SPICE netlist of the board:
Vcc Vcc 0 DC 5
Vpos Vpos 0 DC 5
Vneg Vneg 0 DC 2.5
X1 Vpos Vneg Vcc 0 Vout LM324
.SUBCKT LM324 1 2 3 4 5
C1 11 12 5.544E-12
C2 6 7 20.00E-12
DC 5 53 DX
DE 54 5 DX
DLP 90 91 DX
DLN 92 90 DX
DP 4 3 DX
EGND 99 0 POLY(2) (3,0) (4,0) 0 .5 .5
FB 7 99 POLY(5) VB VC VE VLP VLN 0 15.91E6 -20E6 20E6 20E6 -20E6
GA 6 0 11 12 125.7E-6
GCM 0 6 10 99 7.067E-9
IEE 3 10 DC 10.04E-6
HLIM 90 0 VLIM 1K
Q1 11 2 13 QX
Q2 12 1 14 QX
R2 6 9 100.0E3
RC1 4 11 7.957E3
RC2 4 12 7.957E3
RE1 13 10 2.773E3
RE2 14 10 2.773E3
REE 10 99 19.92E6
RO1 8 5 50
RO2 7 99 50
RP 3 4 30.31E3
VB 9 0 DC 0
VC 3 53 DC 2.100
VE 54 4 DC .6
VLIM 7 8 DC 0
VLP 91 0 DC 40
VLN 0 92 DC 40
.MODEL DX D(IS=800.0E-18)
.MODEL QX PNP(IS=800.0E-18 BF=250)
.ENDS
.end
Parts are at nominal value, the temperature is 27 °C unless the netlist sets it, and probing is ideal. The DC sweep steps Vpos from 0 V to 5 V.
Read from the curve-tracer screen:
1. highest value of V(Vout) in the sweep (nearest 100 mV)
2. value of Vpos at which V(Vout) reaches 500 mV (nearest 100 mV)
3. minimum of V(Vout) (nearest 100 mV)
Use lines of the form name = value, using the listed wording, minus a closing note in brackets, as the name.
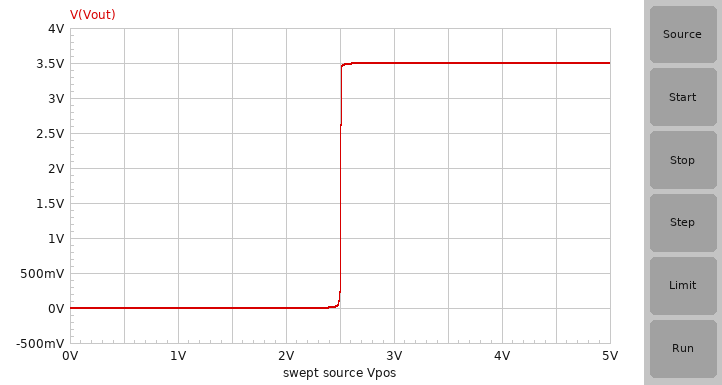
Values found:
highest value of V(Vout) in the sweep = 3.5 V
value of Vpos at which V(Vout) reaches 500 mV = 2.5 V
minimum of V(Vout) = 0 V
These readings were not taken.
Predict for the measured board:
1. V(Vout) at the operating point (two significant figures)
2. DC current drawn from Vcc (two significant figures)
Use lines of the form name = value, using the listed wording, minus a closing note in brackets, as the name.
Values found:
V(Vout) at the operating point = 3.5 V
DC current drawn from Vcc = 170 µA
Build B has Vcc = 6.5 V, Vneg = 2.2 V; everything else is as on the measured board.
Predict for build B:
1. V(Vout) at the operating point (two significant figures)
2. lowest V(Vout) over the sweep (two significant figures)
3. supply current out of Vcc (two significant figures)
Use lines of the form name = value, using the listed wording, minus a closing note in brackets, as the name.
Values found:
V(Vout) at the operating point = 5.0 V
lowest V(Vout) over the sweep = 4.3 mV
supply current out of Vcc = 220 µA
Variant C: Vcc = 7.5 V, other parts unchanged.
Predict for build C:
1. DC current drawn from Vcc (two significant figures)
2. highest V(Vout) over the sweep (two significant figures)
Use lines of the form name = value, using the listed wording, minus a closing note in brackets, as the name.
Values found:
DC current drawn from Vcc = 250 µA
highest V(Vout) over the sweep = 6.0 V
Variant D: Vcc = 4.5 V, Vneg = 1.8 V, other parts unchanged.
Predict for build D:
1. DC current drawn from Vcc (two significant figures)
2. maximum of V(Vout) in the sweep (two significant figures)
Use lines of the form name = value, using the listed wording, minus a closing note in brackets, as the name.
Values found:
DC current drawn from Vcc = 150 µA
maximum of V(Vout) in the sweep = 3.0 V
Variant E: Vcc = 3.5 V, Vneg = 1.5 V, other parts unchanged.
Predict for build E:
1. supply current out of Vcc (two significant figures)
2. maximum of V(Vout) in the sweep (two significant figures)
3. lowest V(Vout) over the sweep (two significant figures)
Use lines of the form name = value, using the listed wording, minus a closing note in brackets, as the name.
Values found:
supply current out of Vcc = 120 µA
maximum of V(Vout) in the sweep = 2.0 V
lowest V(Vout) over the sweep = 4.5 mV
